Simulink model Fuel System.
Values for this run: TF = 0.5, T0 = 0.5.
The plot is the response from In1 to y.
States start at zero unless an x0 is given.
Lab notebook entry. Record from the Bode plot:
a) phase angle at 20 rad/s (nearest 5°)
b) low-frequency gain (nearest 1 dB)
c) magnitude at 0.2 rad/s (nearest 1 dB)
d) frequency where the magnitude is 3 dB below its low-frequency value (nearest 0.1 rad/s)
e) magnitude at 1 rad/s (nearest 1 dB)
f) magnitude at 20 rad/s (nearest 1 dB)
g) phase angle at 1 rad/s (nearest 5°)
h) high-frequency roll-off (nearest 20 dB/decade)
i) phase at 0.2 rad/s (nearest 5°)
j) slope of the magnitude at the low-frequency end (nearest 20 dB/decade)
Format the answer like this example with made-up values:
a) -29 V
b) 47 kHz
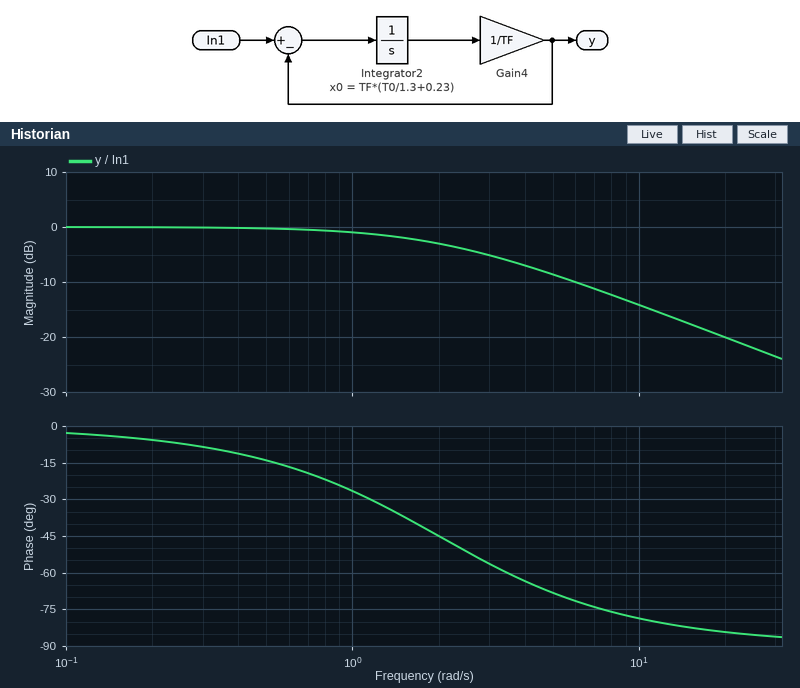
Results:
a) -85°
b) 0 dB
c) 0 dB
d) 2.0 rad/s
e) -1 dB
f) -20 dB
g) -25°
h) -20 dB/decade
i) -5°
j) 0 dB/decade
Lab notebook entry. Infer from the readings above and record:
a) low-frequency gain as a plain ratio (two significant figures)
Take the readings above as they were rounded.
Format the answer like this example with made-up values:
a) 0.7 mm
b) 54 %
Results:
a) 1.0
